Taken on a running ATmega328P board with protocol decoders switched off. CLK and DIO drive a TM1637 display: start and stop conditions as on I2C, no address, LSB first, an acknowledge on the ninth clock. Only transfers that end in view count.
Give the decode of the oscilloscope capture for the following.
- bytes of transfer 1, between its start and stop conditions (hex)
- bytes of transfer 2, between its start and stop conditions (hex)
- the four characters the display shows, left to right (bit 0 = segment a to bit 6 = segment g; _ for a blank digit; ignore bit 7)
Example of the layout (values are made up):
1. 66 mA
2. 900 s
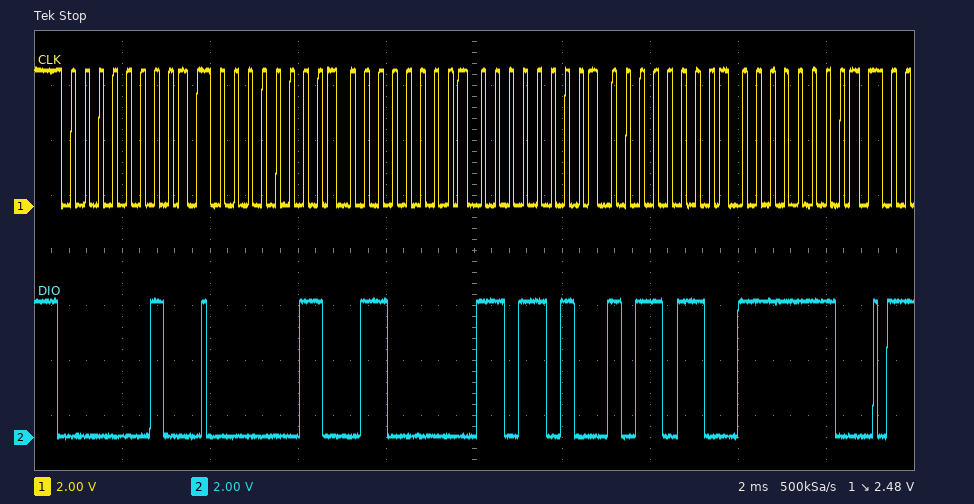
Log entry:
1. 40
2. C0 06 5B 6D 7F
3. 1258
